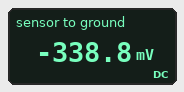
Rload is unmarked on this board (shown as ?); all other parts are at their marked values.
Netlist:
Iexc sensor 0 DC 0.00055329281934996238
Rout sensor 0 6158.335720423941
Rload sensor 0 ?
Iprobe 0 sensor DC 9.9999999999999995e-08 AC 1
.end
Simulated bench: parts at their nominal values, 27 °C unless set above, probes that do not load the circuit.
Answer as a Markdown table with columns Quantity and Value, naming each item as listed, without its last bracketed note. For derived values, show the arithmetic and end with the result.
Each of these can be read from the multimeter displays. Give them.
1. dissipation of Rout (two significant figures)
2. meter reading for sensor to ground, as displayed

| Quantity | Value |
|---|---|
| dissipation of Rout | (0 V - (-338.8 mV))^2 / 6.158 kΩ = 19 µW |
| meter reading for sensor to ground, as displayed | -338.8 mV |
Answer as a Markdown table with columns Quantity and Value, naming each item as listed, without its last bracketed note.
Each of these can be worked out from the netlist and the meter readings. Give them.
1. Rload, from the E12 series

| Quantity | Value |
|---|---|
| Rload, from the E12 series | 680 Ω |
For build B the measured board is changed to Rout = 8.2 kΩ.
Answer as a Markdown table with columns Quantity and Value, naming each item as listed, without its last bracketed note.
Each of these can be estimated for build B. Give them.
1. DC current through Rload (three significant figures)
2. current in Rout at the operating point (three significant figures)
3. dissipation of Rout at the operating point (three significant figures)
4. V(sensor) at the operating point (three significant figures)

| Quantity | Value |
|---|---|
| DC current through Rload | 511 µA |
| current in Rout at the operating point | 42.4 µA |
| dissipation of Rout at the operating point | 14.7 µW |
| V(sensor) at the operating point | -347 mV |
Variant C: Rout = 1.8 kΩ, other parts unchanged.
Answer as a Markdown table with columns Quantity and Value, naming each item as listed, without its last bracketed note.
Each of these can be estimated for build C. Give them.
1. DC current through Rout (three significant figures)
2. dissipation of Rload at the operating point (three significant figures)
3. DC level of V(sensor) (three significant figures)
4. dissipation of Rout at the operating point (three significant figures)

| Quantity | Value |
|---|---|
| DC current through Rout | 152 µA |
| dissipation of Rload at the operating point | 110 µW |
| DC level of V(sensor) | -273 mV |
| dissipation of Rout at the operating point | 41.4 µW |
